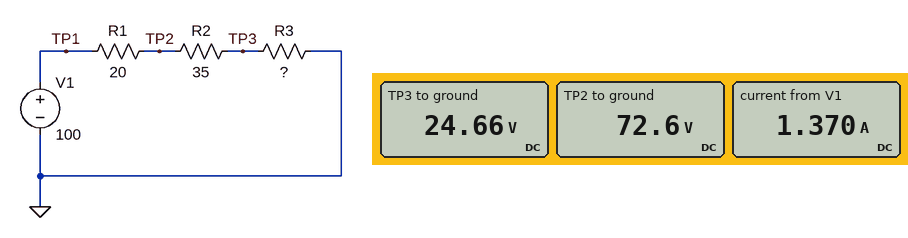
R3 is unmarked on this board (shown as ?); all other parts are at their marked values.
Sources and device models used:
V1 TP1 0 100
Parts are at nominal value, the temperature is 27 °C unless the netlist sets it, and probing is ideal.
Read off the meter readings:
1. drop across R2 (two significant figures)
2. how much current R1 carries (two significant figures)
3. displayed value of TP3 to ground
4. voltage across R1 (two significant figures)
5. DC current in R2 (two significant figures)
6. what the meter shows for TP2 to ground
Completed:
48 V
1.4 A
24.66 V
27 V
1.4 A
72.6 V
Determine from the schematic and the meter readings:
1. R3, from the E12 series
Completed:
18 Ω
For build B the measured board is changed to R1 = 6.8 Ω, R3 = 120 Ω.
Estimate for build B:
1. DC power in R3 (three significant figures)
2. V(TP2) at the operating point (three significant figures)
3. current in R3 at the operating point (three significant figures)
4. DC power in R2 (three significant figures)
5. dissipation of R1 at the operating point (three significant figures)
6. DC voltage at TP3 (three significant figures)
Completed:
45.8 W
95.8 V
618 mA
13.4 W
2.60 W
74.2 V
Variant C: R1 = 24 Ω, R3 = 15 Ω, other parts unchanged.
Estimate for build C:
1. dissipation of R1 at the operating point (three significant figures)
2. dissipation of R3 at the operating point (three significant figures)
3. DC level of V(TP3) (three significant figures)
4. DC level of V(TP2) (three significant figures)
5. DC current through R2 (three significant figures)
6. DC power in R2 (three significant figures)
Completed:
43.8 W
27.4 W
20.3 V
67.6 V
1.35 A
63.9 W
